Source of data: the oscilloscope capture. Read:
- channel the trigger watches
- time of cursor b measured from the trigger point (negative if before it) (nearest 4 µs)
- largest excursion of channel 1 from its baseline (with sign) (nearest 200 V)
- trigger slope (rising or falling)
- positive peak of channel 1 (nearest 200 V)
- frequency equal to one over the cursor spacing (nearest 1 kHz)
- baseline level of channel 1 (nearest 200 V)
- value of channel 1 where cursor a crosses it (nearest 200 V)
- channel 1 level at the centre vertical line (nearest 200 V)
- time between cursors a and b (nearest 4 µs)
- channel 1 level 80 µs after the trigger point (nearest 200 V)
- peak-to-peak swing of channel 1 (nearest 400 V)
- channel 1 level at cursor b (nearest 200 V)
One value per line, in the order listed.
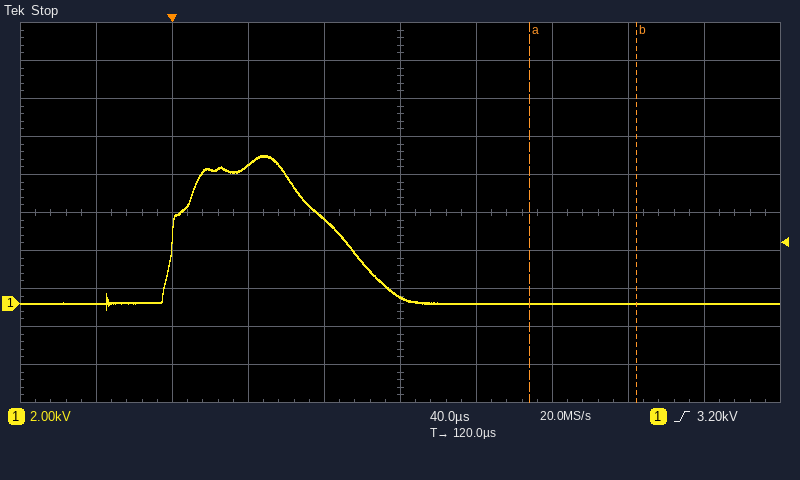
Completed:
channel 1
+244 µs
+7.8 kV
rising
7.8 kV
18 kHz
0.0 kV
0.0 kV
400 V
56 µs
4.4 kV
8.0 kV
0.0 kV
